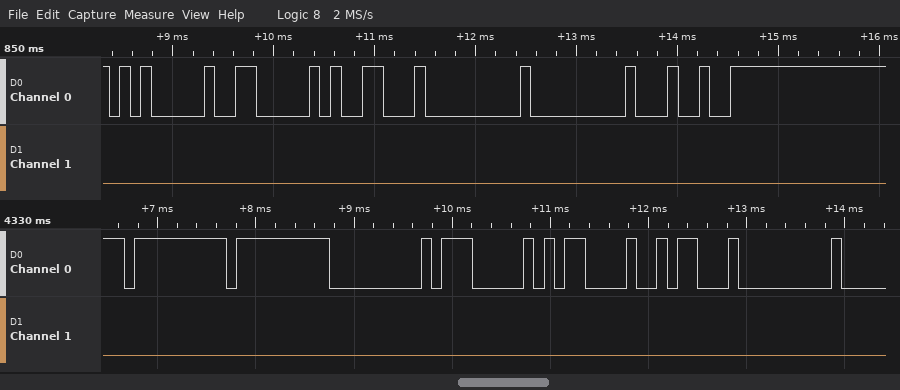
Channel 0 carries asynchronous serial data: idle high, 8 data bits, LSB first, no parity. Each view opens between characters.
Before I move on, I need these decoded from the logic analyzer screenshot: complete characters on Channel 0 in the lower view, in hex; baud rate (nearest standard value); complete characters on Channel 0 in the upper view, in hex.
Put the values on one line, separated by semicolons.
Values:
FF, FF, 00, 07, 0D, 1A, 00; 9600 baud; 05, 06, 19, 00, 00, 24
